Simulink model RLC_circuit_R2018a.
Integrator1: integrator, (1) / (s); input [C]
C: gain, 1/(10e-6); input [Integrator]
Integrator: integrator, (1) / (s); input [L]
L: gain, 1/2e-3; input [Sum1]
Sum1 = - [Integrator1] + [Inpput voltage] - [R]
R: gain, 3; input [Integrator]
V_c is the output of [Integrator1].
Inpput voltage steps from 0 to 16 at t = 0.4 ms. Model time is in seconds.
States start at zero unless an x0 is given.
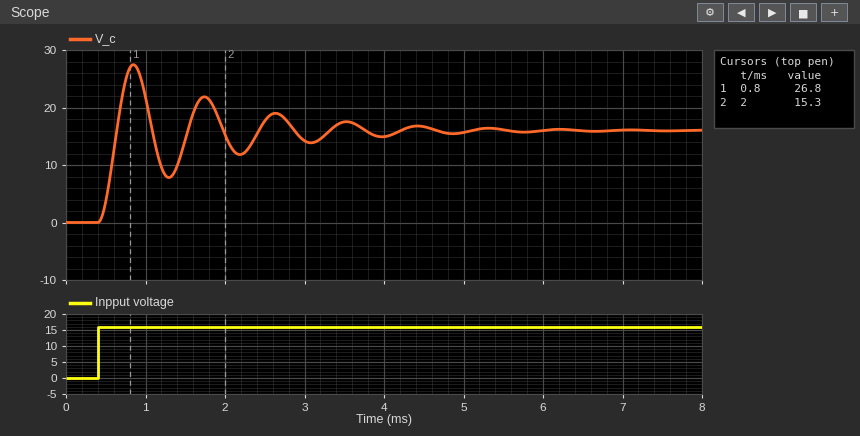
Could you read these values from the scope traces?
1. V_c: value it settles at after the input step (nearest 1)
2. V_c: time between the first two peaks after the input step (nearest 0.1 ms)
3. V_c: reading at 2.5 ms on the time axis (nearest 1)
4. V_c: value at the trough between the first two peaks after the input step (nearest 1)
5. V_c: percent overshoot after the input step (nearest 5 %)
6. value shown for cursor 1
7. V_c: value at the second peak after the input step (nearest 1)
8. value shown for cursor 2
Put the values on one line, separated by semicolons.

16; 0.9 ms; 18; 8; 70 %; 26.8; 22; 15.3
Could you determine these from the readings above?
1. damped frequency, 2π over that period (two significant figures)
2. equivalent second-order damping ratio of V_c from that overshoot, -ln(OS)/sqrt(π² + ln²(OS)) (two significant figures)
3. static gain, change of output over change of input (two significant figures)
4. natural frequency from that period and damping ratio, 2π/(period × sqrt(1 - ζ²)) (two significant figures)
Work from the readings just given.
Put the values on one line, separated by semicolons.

7.0 rad/ms; 0.11; 1.0; 7.0 rad/ms
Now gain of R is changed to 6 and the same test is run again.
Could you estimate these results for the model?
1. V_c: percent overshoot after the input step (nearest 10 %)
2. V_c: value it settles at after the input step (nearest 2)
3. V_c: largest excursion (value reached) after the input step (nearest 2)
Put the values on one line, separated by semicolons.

50 %; 16; 24
